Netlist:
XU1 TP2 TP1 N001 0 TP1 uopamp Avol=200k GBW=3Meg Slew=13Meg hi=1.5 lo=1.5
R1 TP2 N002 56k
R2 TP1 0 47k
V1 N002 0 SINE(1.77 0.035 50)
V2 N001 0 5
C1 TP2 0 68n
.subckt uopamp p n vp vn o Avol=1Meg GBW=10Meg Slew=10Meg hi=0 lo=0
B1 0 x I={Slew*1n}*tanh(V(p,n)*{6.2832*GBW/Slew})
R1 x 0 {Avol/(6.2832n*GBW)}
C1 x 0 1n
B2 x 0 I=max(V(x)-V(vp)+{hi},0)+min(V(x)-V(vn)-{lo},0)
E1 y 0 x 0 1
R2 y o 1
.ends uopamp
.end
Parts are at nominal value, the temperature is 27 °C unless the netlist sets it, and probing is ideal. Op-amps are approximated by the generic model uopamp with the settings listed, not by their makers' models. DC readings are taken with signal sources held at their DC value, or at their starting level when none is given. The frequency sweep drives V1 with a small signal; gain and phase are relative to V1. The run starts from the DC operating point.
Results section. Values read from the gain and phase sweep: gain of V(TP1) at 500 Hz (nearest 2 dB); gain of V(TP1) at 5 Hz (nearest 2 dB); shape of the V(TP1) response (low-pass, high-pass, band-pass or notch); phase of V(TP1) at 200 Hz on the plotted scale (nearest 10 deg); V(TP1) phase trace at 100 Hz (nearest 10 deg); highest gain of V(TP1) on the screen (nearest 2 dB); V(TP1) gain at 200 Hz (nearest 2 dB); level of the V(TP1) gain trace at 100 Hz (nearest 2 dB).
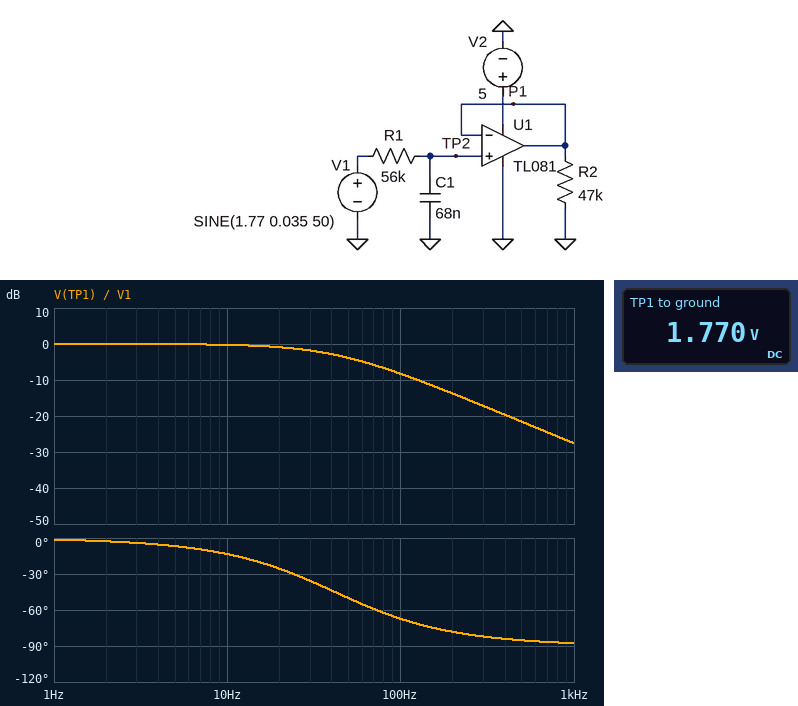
-22 dB
0 dB
low-pass
-80 deg
-70 deg
0 dB
-14 dB
-8 dB
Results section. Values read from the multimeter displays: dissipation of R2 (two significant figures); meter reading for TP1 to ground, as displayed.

67 µW
1.770 V
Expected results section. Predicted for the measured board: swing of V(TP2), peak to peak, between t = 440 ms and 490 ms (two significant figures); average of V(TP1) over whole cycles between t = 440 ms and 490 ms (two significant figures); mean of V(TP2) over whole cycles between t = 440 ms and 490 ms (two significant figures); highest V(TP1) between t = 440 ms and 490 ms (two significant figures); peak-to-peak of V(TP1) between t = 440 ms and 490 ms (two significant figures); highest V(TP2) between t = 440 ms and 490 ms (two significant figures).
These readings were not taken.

45 mV
1.8 V
1.8 V
1.8 V
45 mV
1.8 V
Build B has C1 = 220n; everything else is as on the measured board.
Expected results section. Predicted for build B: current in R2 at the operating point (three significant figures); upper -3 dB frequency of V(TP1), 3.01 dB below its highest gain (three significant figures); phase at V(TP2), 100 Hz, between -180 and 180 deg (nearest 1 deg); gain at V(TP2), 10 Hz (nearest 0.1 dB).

37.7 µA
12.9 Hz
-83 deg
-2.0 dB
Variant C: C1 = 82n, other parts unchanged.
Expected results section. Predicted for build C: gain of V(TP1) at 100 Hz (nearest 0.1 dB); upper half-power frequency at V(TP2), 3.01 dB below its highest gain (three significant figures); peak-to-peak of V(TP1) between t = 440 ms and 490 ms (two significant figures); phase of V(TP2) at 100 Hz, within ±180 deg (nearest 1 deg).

-9.7 dB
34.7 Hz
40 mV
-71 deg
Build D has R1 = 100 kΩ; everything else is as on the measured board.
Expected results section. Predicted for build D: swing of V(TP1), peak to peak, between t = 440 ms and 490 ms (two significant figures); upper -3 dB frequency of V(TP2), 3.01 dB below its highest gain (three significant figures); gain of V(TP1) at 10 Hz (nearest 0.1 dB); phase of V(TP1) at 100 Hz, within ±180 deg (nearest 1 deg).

30 mV
23.4 Hz
-0.7 dB
-77 deg
